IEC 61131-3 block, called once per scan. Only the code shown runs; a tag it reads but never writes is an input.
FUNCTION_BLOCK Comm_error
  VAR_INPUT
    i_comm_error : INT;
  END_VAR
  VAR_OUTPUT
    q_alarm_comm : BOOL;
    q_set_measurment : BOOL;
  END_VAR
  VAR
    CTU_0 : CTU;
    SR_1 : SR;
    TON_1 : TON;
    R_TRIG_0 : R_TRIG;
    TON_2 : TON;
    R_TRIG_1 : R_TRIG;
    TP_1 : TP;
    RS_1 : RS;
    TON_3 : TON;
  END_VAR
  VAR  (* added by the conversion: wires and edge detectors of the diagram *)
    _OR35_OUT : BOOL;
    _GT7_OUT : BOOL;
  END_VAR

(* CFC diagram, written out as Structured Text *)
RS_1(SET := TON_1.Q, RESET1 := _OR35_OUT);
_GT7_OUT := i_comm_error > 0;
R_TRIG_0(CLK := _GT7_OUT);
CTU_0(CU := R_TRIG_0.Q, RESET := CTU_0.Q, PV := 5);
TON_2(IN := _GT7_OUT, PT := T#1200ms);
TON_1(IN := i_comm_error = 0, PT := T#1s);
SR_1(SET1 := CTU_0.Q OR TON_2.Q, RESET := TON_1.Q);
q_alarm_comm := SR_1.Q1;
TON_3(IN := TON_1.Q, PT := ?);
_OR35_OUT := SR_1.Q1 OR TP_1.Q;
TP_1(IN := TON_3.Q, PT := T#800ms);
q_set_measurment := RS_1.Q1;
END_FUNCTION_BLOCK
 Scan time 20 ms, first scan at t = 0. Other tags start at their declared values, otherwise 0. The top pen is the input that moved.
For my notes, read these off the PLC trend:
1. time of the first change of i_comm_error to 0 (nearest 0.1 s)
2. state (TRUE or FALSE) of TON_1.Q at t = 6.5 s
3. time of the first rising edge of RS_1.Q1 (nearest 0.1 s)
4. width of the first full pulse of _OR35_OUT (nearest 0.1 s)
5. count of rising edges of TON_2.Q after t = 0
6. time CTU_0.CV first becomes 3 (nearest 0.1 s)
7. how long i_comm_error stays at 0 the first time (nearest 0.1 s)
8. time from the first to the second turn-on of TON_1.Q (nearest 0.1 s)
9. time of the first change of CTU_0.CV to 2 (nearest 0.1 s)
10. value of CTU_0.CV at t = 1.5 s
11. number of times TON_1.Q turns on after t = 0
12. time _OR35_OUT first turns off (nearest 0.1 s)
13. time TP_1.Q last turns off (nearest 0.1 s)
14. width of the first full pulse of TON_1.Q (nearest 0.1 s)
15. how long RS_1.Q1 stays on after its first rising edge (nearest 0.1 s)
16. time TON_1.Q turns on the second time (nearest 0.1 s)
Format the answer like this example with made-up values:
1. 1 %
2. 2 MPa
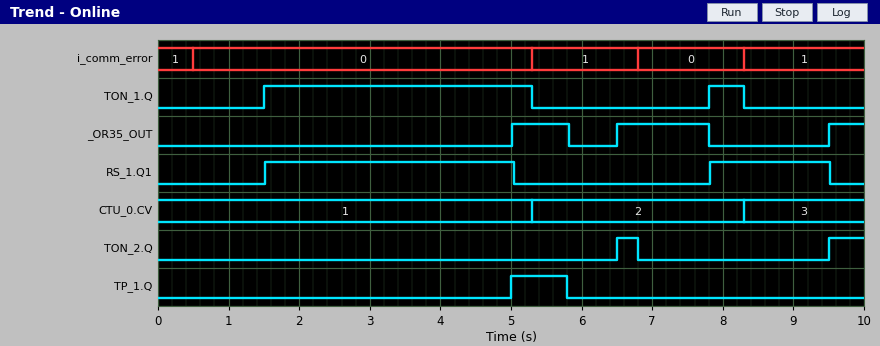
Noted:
1. 0.5 s
2. FALSE
3. 1.5 s
4. 0.8 s
5. 2
6. 8.3 s
7. 4.8 s
8. 6.3 s
9. 5.3 s
10. 1
11. 2
12. 5.8 s
13. 5.8 s
14. 3.8 s
15. 3.5 s
16. 7.8 s
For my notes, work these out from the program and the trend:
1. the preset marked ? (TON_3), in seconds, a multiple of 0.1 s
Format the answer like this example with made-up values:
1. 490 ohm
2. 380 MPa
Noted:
1. 3.5 s
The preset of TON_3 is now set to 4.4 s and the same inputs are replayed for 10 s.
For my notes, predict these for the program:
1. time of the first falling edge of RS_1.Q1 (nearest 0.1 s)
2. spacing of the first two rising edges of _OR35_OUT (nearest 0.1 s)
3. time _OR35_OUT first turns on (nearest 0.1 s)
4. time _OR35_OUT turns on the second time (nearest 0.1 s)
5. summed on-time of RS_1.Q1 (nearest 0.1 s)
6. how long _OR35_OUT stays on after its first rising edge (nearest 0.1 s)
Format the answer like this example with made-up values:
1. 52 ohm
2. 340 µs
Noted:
1. 6.5 s
2. 3.0 s
3. 6.5 s
4. 9.5 s
5. 6.7 s
6. 1.3 s
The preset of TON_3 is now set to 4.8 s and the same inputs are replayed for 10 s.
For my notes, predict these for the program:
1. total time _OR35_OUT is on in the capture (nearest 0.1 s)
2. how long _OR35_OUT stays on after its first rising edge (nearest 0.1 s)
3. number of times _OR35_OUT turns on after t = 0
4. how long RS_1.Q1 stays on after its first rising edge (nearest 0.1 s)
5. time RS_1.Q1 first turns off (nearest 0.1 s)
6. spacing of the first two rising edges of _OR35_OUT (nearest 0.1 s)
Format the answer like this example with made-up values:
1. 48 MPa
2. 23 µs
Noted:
1. 1.8 s
2. 1.3 s
3. 2
4. 5.0 s
5. 6.5 s
6. 3.0 s
